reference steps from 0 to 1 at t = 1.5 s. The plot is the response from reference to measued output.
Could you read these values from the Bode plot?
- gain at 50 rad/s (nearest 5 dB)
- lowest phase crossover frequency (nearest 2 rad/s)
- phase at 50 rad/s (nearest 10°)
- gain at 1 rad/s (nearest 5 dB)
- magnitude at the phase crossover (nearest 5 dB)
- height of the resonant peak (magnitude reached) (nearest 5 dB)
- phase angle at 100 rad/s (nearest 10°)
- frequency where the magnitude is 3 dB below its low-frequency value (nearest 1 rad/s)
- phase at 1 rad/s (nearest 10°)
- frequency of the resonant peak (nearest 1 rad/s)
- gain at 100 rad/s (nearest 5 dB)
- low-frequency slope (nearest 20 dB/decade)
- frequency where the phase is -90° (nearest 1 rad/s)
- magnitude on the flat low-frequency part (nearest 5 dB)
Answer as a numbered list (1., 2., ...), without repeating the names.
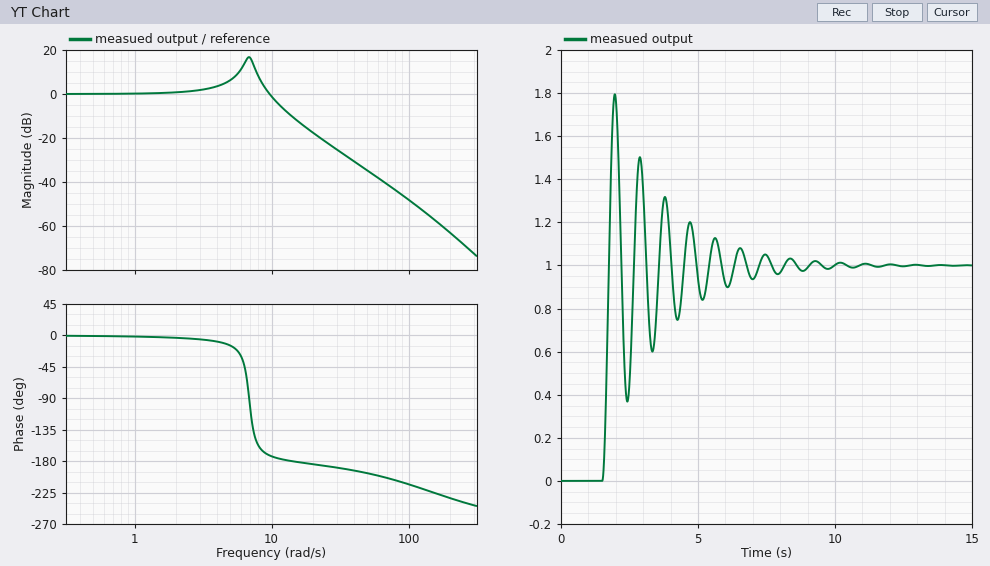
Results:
1. -35 dB
2. 14 rad/s
3. -200°
4. 0 dB
5. -10 dB
6. 15 dB
7. -210°
8. 11 rad/s
9. 0°
10. 7 rad/s
11. -50 dB
12. 0 dB/decade
13. 7 rad/s
14. 0 dB
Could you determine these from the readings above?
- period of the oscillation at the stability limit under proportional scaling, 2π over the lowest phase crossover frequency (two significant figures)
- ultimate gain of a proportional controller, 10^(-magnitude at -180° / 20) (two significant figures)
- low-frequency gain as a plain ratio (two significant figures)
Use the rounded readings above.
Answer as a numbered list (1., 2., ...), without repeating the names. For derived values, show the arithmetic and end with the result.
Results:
1. 2π / 14 = 0.45 s
2. 10^(10 / 20) = 3.2
3. 10^(0 / 20) = 1.0
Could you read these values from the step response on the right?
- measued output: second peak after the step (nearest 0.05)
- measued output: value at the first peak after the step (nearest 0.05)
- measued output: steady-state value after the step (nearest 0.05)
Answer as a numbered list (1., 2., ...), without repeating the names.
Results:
1. 1.50
2. 1.80
3. 1.00
